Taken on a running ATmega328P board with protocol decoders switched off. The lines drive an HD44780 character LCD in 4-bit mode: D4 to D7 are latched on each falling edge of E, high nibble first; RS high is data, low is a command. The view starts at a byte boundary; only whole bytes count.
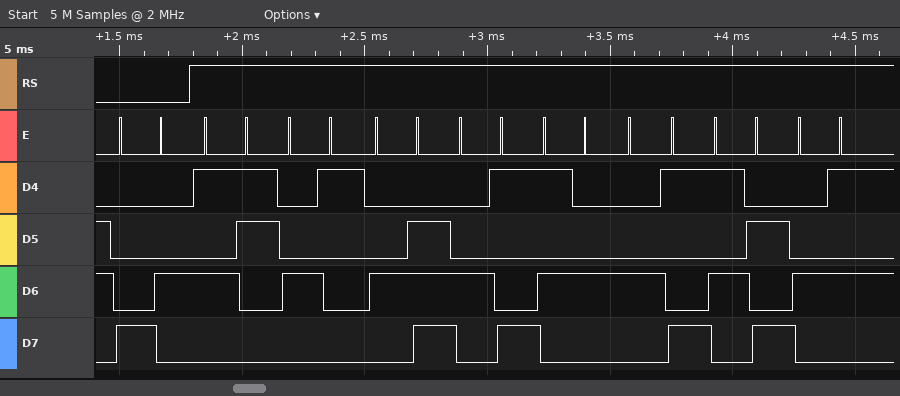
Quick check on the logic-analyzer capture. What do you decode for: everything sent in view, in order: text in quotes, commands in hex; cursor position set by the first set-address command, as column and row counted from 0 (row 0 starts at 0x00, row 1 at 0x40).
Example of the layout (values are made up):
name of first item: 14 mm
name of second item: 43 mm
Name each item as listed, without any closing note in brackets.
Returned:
everything sent in view, in order: text in quotes, commands in hex: 0x84 "SANITIZE"
cursor position set by the first set-address command, as column and row counted from 0: column 4, row 0
